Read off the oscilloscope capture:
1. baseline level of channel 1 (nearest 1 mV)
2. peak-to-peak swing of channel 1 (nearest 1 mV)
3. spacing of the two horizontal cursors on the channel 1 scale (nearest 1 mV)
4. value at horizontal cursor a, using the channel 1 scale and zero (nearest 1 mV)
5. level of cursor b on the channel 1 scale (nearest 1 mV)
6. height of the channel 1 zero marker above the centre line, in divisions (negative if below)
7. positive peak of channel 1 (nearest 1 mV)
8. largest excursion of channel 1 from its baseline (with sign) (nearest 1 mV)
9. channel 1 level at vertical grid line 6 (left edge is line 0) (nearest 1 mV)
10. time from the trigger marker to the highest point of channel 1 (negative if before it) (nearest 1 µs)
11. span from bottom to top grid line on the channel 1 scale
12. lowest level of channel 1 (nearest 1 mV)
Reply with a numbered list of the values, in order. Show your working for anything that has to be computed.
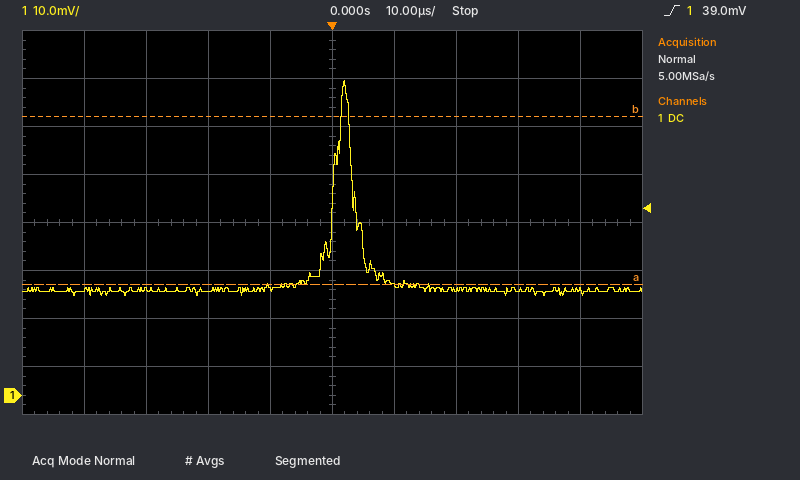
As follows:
1. 22 mV
2. 66 mV − (21 mV) = 45 mV
3. 35 mV
4. 23 mV
5. 58 mV
6. -3.6 div
7. 66 mV
8. 66 mV − (22 mV) = +44 mV
9. 23 mV
10. +2 µs
11. 80 mV
12. 21 mV
